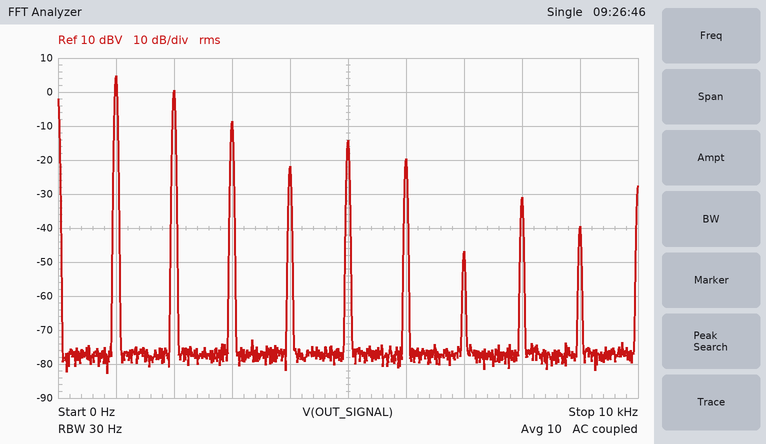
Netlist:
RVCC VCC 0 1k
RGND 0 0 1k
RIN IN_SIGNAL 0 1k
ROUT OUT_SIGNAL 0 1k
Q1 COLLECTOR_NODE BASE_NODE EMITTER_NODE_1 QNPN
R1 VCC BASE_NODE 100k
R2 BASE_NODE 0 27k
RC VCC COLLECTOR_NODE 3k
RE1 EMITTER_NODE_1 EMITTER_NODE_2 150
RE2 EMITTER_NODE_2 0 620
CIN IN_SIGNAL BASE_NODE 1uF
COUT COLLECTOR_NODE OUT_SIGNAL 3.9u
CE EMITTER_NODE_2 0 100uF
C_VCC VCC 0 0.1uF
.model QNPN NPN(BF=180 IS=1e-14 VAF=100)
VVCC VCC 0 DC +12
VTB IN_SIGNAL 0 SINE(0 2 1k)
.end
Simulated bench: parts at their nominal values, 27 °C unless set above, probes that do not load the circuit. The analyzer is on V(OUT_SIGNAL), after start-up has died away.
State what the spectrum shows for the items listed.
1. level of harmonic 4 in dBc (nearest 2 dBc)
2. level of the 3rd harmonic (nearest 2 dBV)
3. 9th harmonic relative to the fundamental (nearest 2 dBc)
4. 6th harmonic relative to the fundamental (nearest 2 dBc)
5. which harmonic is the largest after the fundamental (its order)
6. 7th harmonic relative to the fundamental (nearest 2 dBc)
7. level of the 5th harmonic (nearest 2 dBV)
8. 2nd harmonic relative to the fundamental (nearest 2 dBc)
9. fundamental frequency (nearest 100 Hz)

-26 dBc
-8 dBV
-44 dBc
-24 dBc
2
-52 dBc
-14 dBV
-4 dBc
1.0 kHz
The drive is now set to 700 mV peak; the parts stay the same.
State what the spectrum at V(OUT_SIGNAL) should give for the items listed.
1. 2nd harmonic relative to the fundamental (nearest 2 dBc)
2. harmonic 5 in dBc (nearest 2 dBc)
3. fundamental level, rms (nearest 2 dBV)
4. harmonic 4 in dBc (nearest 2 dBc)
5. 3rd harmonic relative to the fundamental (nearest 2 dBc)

-12 dBc
-32 dBc
4 dBV
-40 dBc
-22 dBc
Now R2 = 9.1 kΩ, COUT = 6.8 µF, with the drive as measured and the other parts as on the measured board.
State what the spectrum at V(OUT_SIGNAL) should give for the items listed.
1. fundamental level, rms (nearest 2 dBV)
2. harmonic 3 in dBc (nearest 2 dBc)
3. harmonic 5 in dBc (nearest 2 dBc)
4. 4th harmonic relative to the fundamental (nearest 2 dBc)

4 dBV
-12 dBc
-22 dBc
-44 dBc
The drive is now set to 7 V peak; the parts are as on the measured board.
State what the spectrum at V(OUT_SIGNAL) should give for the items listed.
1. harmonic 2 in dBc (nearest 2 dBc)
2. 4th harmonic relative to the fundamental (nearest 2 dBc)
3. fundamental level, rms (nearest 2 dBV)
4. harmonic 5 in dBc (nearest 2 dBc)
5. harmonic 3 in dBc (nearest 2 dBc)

-2 dBc
-10 dBc
4 dBV
-22 dBc
-4 dBc
